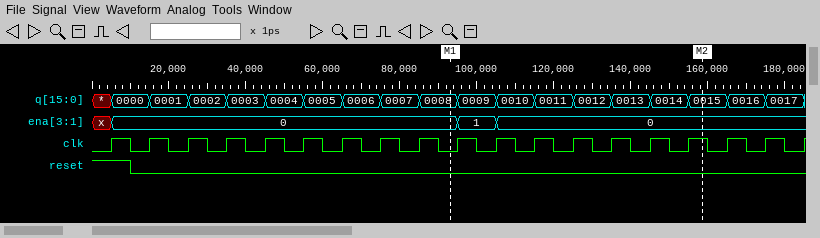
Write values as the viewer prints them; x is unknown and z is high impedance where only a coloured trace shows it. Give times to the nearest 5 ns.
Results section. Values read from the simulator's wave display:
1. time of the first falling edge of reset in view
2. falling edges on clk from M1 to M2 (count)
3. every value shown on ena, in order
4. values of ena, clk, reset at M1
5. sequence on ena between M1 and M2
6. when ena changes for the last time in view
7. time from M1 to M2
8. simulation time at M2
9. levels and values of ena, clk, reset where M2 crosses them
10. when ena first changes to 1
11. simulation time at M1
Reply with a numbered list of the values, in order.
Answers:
1. 10 ns
2. 6
3. x, 0, 1, 0
4. ena=0, clk=0, reset=0
5. 0, 1, 0
6. 105 ns
7. 65 ns
8. 160 ns
9. ena=0, clk=1, reset=0
10. 95 ns
11. 95 ns
